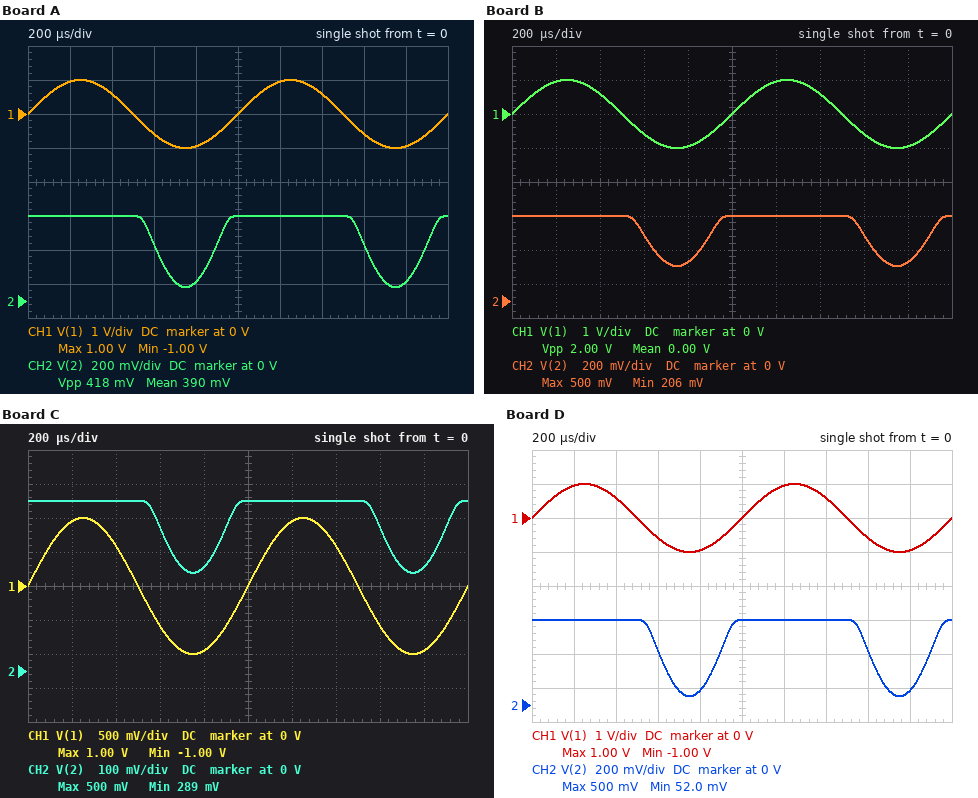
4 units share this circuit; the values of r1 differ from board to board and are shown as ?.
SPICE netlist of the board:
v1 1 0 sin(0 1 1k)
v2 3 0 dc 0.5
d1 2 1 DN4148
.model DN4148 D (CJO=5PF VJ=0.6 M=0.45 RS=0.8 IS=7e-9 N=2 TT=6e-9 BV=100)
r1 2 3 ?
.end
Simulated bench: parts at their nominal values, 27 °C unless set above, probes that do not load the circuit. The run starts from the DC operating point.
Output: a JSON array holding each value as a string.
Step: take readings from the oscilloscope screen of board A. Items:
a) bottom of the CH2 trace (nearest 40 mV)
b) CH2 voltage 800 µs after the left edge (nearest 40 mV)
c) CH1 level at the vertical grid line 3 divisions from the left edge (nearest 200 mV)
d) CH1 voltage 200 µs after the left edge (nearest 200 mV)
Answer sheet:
["80 mV", "120 mV", "-600 mV", "1.0 V"]
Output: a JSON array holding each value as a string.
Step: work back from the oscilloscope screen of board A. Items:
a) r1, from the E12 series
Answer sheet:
["1.8 Ω"]
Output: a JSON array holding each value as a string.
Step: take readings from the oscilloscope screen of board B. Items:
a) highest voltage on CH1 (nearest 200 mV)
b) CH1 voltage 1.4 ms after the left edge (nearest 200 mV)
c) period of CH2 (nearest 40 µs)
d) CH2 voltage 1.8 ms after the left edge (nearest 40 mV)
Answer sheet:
["1.0 V", "600 mV", "1.00 ms", "240 mV"]
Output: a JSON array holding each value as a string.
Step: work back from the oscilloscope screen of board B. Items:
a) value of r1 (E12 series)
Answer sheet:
["0.82 Ω"]
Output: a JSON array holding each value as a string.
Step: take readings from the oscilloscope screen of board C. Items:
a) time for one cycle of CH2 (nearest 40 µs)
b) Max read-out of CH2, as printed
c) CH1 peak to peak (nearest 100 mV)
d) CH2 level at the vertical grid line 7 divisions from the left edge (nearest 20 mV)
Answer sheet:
["1.00 ms", "500 mV", "2.0 V", "500 mV"]
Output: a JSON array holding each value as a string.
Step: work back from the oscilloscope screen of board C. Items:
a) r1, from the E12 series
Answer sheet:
["0.47 Ω"]
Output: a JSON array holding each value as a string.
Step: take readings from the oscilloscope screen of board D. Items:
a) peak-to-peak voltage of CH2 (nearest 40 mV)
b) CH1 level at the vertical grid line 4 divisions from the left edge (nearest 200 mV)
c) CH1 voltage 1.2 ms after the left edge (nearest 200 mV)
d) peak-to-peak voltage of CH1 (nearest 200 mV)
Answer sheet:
["440 mV", "-1.0 V", "1.0 V", "2.0 V"]
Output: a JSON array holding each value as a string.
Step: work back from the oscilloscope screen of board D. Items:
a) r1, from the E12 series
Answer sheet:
["2.2 Ω"]
